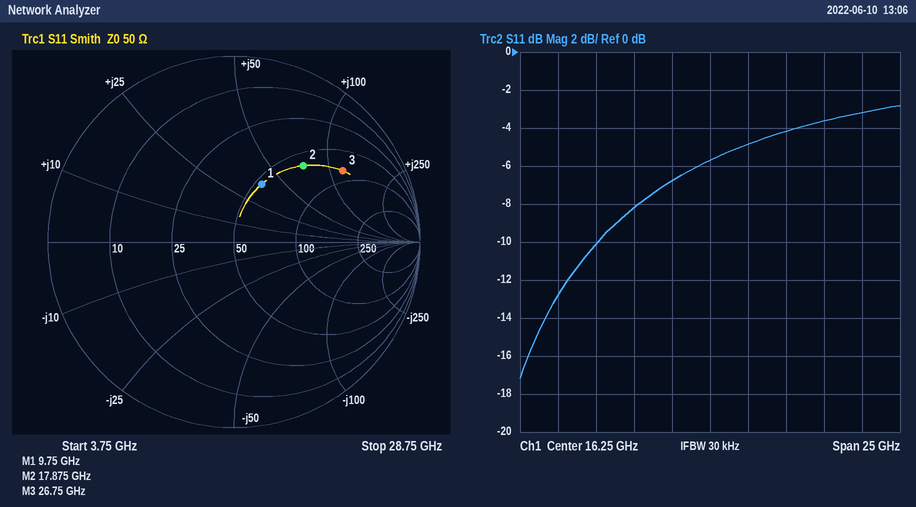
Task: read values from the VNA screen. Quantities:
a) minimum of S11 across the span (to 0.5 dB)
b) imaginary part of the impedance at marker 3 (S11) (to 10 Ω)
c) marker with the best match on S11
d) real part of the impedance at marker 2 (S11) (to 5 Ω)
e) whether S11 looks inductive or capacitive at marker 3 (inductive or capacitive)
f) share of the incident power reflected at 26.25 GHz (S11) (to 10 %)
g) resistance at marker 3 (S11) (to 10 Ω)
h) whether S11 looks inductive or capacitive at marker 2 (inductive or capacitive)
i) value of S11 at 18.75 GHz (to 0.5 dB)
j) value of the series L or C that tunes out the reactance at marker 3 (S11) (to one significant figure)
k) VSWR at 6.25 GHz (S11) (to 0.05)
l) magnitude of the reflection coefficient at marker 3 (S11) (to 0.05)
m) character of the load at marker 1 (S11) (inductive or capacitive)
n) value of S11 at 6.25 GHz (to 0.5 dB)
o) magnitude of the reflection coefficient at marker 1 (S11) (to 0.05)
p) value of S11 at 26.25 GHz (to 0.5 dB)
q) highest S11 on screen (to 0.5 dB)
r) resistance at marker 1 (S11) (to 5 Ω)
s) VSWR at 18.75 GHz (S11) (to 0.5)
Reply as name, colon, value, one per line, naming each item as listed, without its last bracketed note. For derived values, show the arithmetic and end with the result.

minimum of S11 across the span: -17.0 dB
imaginary part of the impedance at marker 3 (S11): +120 Ω
marker with the best match on S11: marker 1
real part of the impedance at marker 2 (S11): 60 Ω
whether S11 looks inductive or capacitive at marker 3: inductive
share of the incident power reflected at 26.25 GHz (S11): 10^(-3/10) ≈ 50 %
resistance at marker 3 (S11): 80 Ω
whether S11 looks inductive or capacitive at marker 2: inductive
value of S11 at 18.75 GHz: -5.0 dB
value of the series L or C that tunes out the reactance at marker 3 (S11): C = 1/(2π × 26.75 GHz × 120 Ω) ≈ 50 fF
VSWR at 6.25 GHz (S11): |Γ| = 10^(-13/20) = 0.2239; VSWR = (1 + 0.2239)/(1 − 0.2239) ≈ 1.58, so 1.60 to the nearest 0.05
magnitude of the reflection coefficient at marker 3 (S11): 0.70
character of the load at marker 1 (S11): inductive
value of S11 at 6.25 GHz: -13.0 dB
magnitude of the reflection coefficient at marker 1 (S11): 0.35
value of S11 at 26.25 GHz: -3.0 dB
highest S11 on screen: -3.0 dB
resistance at marker 1 (S11): 55 Ω
VSWR at 18.75 GHz (S11): |Γ| = 10^(-5/20) = 0.5623; VSWR = (1 + 0.5623)/(1 − 0.5623) ≈ 3.57, so 3.5 to the nearest 0.5
